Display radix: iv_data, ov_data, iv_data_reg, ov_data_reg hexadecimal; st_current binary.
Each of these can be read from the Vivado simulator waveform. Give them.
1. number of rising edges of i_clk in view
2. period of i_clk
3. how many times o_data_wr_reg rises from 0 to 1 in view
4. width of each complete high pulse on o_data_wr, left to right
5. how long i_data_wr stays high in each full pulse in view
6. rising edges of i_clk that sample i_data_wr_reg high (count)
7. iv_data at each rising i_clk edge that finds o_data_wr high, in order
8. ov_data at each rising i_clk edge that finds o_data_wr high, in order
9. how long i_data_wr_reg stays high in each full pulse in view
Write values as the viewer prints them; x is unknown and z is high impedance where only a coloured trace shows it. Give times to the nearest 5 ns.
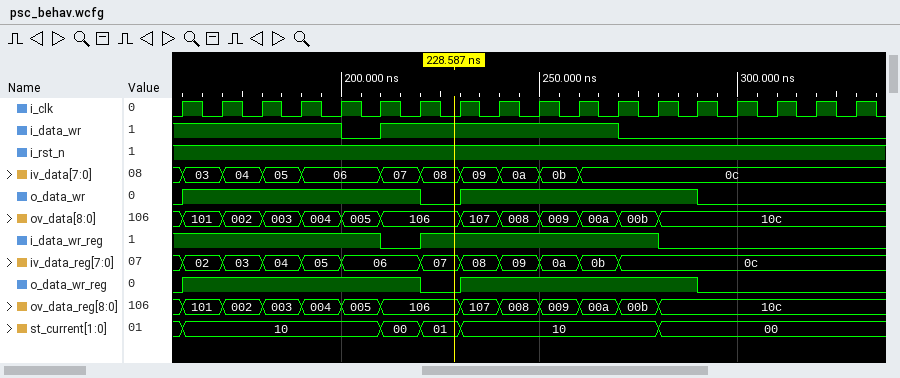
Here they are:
18
10 ns
2
60 ns, 60 ns
60 ns
12
03, 04, 05, 06, 06, 07, 09, 0a, 0b, 0c, 0c, 0c
101, 002, 003, 004, 005, 106, 107, 008, 009, 00a, 00b, 10c
60 ns
